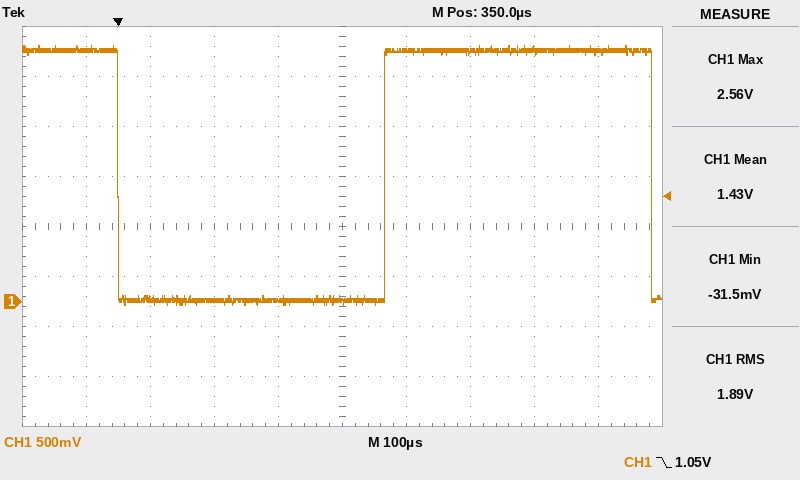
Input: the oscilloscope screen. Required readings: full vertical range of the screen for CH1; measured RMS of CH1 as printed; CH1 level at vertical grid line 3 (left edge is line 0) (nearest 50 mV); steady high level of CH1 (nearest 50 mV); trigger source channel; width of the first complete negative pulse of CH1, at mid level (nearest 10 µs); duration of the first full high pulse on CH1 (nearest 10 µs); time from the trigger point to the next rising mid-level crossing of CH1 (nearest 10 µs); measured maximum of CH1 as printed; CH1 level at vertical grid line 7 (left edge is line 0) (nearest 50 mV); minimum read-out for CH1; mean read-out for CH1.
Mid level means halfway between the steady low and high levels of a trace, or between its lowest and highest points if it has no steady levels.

4 V
1.89 V
0 mV
2.50 V
CH1
420 µs
420 µs
420 µs
2.56 V
2.50 V
-31.5 mV
1.43 V
